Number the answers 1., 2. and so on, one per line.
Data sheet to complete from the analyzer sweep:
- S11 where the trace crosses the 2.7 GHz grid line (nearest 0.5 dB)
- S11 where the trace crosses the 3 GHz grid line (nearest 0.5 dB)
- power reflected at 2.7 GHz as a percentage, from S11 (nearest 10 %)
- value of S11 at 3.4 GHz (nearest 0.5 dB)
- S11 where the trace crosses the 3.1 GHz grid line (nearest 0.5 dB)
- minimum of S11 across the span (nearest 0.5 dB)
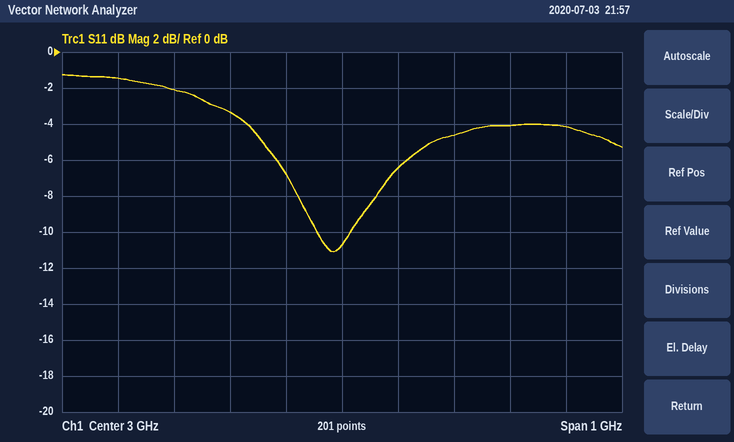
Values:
1. -2.0 dB
2. -10.5 dB
3. 60 %
4. -4.0 dB
5. -6.5 dB
6. -11.0 dB
